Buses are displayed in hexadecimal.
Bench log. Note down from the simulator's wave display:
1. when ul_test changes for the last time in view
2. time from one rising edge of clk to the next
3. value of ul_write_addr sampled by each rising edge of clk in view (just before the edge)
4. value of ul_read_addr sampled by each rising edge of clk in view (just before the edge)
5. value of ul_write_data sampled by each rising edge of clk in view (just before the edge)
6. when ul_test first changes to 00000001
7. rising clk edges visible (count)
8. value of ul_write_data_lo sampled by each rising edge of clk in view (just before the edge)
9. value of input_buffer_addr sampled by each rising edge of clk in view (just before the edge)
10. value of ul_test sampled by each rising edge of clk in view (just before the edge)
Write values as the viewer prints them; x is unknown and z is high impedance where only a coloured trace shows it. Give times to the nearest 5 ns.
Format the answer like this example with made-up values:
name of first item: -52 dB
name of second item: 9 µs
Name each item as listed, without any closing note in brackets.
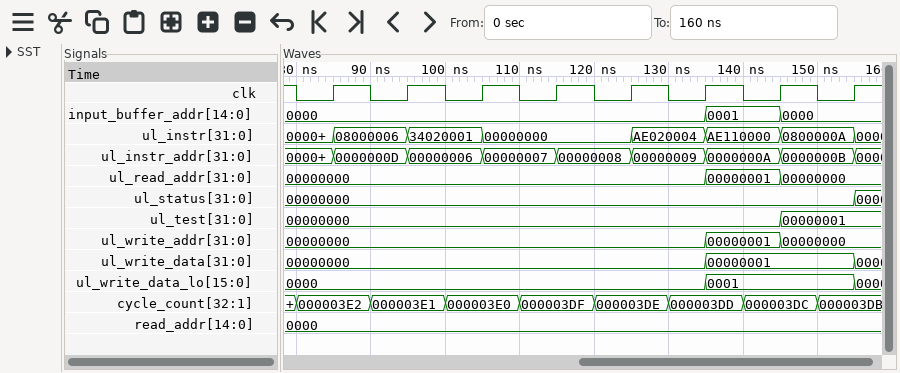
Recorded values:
when ul_test changes for the last time in view: 145 ns
time from one rising edge of clk to the next: 10 ns
value of ul_write_addr sampled by each rising edge of clk in view: 00000000, 00000000, 00000000, 00000000, 00000000, 00000000, 00000001, 00000000
value of ul_read_addr sampled by each rising edge of clk in view: 00000000, 00000000, 00000000, 00000000, 00000000, 00000000, 00000001, 00000000
value of ul_write_data sampled by each rising edge of clk in view: 00000000, 00000000, 00000000, 00000000, 00000000, 00000000, 00000001, 00000001
when ul_test first changes to 00000001: 145 ns
rising clk edges visible: 8
value of ul_write_data_lo sampled by each rising edge of clk in view: 0000, 0000, 0000, 0000, 0000, 0000, 0001, 0001
value of input_buffer_addr sampled by each rising edge of clk in view: 0000, 0000, 0000, 0000, 0000, 0000, 0001, 0000
value of ul_test sampled by each rising edge of clk in view: 00000000, 00000000, 00000000, 00000000, 00000000, 00000000, 00000000, 00000001
